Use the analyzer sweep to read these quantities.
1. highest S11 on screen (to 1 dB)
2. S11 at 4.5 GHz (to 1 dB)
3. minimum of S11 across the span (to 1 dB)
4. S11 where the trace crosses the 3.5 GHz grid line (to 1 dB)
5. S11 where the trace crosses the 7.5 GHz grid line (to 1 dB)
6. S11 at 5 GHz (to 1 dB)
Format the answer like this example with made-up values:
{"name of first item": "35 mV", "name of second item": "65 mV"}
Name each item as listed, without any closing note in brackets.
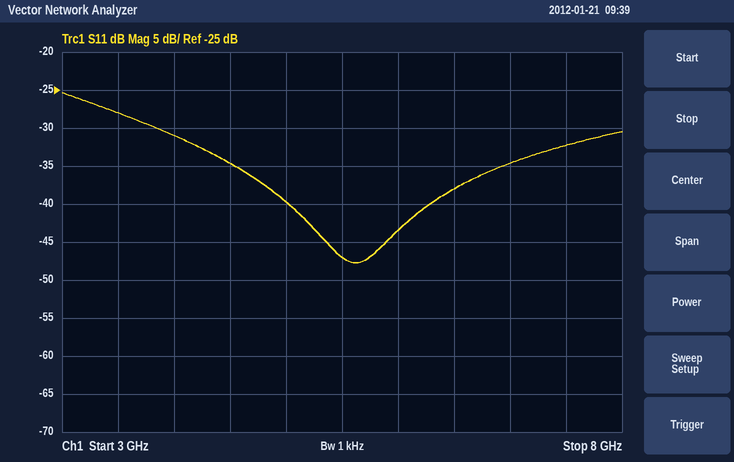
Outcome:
{"highest S11 on screen": "-25 dB", "S11 at 4.5 GHz": "-35 dB", "minimum of S11 across the span": "-48 dB", "S11 where the trace crosses the 3.5 GHz grid line": "-28 dB", "S11 where the trace crosses the 7.5 GHz grid line": "-32 dB", "S11 at 5 GHz": "-40 dB"}
